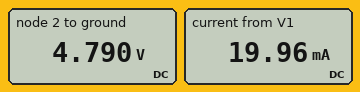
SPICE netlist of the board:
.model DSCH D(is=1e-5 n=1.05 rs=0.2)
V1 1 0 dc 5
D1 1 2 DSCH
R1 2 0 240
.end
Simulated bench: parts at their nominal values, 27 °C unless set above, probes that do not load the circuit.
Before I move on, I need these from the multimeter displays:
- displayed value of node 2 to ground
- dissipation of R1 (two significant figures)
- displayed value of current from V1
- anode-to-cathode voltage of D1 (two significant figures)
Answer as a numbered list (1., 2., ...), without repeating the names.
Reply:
1. 4.790 V
2. 96 mW
3. 19.96 mA
4. 210 mV
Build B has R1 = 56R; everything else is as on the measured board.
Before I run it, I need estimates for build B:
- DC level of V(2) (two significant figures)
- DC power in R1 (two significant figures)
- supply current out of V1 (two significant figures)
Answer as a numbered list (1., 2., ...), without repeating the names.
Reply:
1. 4.7 V
2. 400 mW
3. 85 mA
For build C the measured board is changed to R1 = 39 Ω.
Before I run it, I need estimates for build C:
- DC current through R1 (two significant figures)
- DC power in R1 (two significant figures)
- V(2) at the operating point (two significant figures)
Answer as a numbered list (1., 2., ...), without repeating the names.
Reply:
1. 120 mA
2. 570 mW
3. 4.7 V
